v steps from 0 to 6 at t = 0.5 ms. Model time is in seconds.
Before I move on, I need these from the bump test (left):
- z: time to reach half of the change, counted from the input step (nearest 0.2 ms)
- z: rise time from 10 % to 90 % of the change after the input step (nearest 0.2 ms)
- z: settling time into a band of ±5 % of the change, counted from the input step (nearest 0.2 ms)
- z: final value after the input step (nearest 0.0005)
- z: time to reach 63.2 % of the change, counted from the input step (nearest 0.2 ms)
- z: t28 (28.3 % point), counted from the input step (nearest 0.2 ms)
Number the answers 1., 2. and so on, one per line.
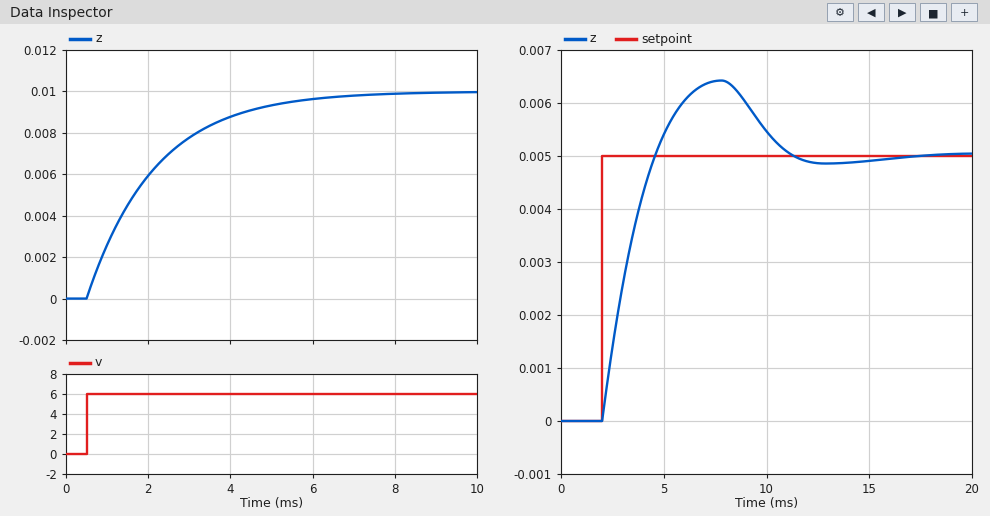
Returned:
1. 1.2 ms
2. 3.6 ms
3. 5.0 ms
4. 0.0100
5. 1.6 ms
6. 0.6 ms
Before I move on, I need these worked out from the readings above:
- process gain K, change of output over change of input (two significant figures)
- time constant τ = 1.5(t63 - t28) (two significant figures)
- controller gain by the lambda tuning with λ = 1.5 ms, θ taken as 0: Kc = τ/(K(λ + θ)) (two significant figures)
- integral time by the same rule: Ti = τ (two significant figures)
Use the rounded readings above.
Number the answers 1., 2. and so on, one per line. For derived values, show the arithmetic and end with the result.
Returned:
1. (0.01 - 0) / 6 = 0.0017
2. 1.5 × (1.6 - 0.6) = 1.5 ms
3. 1.5 / (0.0017 × (1.5 + 0)) = 590
4. 1.5 ms
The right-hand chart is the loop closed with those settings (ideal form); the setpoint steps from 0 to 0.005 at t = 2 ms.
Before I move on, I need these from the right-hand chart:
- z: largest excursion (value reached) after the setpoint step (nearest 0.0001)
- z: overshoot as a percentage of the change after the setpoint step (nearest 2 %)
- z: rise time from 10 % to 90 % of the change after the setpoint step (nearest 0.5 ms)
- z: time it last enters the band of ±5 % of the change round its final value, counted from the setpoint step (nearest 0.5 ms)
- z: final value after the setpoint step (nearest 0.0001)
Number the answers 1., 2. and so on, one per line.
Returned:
1. 0.0064
2. 28 %
3. 2.0 ms
4. 8.5 ms
5. 0.0050
